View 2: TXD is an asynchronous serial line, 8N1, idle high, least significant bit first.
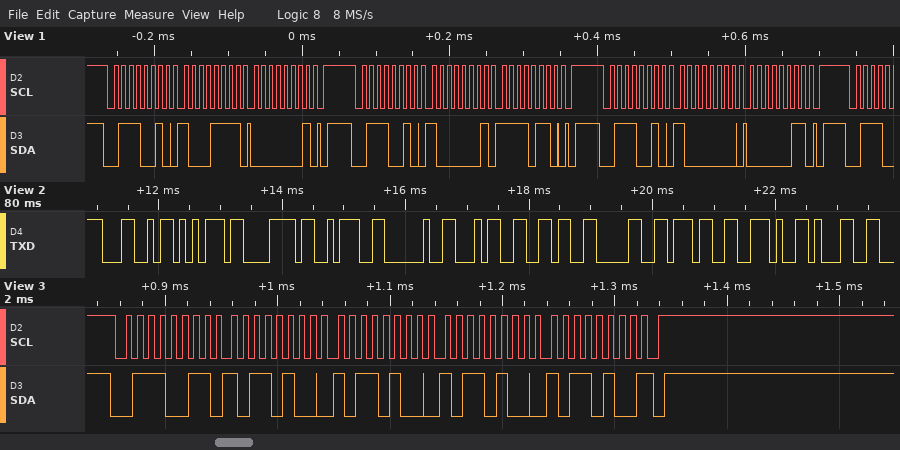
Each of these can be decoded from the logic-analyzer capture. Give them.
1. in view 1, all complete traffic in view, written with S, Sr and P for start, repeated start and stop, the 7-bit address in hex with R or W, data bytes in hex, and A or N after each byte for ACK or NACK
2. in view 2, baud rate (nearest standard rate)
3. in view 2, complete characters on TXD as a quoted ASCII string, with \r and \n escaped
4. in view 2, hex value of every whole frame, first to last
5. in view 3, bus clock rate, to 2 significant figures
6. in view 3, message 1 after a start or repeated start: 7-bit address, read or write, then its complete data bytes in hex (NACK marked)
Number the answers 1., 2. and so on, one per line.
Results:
1. S 39W A 8F A 01 A P S 39W A 81 A F6 A P S 39W A 80 A 03 A P
2. 9600 baud
3. "Lux: 4607.1"
4. 0x4C 0x75 0x78 0x3A 0x20 0x34 0x36 0x30 0x37 0x2E 0x31
5. 100 kHz
6. 0x39 read: B4 B4 B4 B4 NACK
